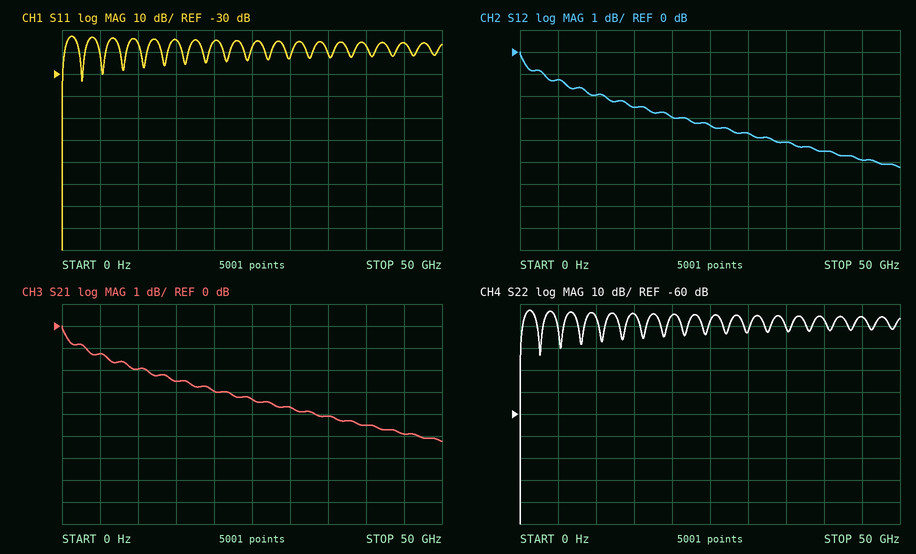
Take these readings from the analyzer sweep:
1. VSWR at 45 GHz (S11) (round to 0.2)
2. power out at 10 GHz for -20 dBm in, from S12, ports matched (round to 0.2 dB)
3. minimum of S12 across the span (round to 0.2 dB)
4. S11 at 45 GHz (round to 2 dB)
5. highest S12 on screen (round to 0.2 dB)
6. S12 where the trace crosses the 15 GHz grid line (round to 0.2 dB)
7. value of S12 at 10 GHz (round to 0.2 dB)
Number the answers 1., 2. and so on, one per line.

1. 1.4
2. -22.0 dBm
3. -5.2 dB
4. -16 dB
5. 0.0 dB
6. -2.6 dB
7. -2.0 dB
